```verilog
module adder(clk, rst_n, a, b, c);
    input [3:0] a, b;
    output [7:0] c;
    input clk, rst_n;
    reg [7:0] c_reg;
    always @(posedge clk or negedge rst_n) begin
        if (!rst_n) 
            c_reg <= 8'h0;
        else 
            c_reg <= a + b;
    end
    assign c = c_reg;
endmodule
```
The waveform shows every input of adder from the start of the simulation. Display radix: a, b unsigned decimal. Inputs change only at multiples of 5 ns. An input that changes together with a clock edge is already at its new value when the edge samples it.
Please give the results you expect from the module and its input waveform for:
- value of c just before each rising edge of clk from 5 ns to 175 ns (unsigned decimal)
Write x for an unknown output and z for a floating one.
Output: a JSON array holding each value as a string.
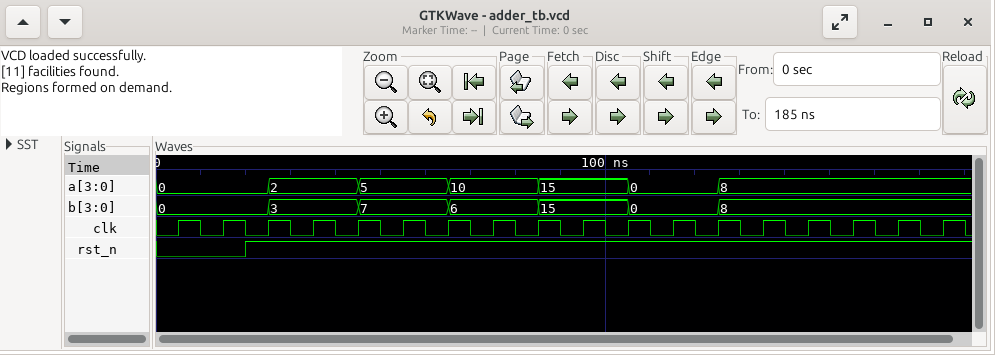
["0, 0, 0, 5, 5, 12, 12, 16, 16, 30, 30, 0, 0, 16, 16, 16, 16, 16"]
